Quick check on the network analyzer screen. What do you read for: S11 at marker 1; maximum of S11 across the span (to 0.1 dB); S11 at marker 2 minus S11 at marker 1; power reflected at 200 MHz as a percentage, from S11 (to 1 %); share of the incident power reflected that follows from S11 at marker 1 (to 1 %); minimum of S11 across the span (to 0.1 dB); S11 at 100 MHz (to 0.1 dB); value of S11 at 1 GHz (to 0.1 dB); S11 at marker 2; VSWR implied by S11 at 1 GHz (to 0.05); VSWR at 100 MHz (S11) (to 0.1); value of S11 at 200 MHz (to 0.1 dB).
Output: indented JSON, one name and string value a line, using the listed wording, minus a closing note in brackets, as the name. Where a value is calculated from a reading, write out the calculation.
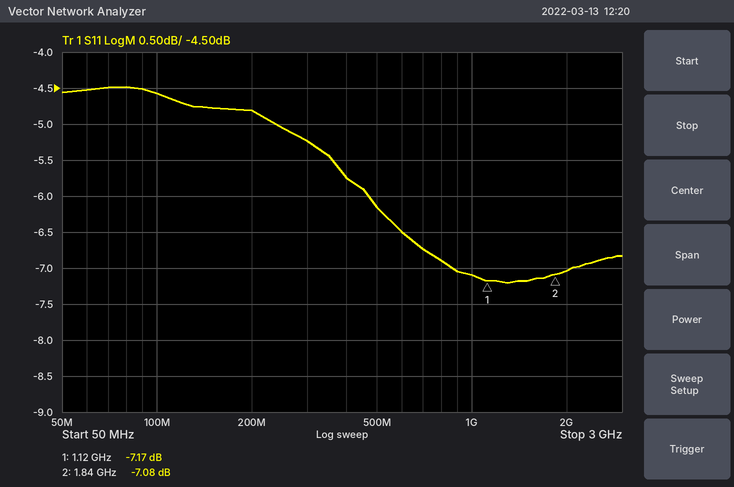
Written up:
{
  "S11 at marker 1": "-7.17 dB",
  "maximum of S11 across the span": "-4.5 dB",
  "S11 at marker 2 minus S11 at marker 1": "-7.08 − (-7.17) = 0.09 dB",
  "power reflected at 200 MHz as a percentage, from S11": "10^(-4.8/10) ≈ 33 %",
  "share of the incident power reflected that follows from S11 at marker 1": "10^(-7.17/10) ≈ 19 %",
  "minimum of S11 across the span": "-7.2 dB",
  "S11 at 100 MHz": "-4.6 dB",
  "value of S11 at 1 GHz": "-7.1 dB",
  "S11 at marker 2": "-7.08 dB",
  "VSWR implied by S11 at 1 GHz": "|Γ| = 10^(-7.1/20) = 0.4416; VSWR = (1 + 0.4416)/(1 − 0.4416) ≈ 2.58, so 2.60 to the nearest 0.05",
  "VSWR at 100 MHz (S11)": "|Γ| = 10^(-4.6/20) = 0.5888; VSWR = (1 + 0.5888)/(1 − 0.5888) ≈ 3.9",
  "value of S11 at 200 MHz": "-4.8 dB"
}
